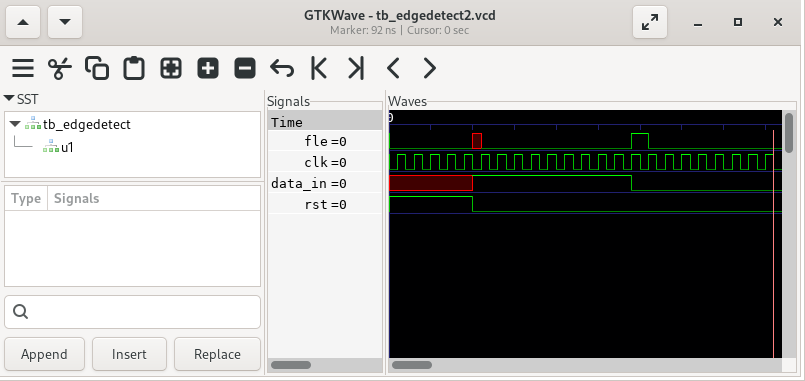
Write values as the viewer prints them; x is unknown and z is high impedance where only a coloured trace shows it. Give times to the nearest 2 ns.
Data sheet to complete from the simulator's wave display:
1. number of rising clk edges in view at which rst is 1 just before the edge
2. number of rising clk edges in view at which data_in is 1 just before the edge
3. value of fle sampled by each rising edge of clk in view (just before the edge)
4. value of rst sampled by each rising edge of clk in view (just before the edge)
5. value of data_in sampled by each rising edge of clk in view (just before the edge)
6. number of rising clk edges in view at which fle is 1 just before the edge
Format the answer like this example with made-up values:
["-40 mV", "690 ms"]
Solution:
["5", "10", "0 0 0 0 0 x 0 0 0 0 0 0 0 0 0 1 0 0 0 0 0 0 0", "1 1 1 1 1 0 0 0 0 0 0 0 0 0 0 0 0 0 0 0 0 0 0", "x x x x x 1 1 1 1 1 1 1 1 1 1 0 0 0 0 0 0 0 0", "1"]
